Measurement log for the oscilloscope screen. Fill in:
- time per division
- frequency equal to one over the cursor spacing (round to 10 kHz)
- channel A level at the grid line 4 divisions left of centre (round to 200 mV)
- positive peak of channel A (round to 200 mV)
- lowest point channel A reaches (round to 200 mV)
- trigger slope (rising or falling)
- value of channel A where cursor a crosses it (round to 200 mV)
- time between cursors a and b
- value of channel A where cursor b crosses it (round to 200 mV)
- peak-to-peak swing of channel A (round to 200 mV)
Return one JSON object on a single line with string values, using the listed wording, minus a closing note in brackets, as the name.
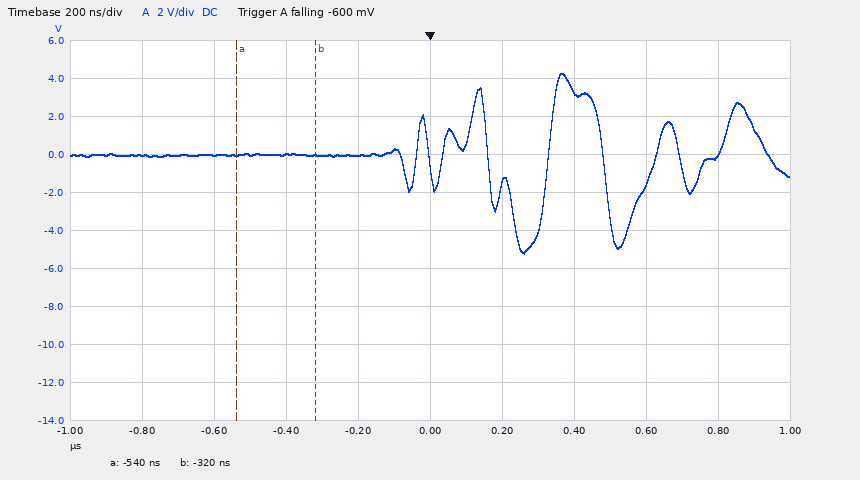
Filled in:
{"time per division": "200 ns", "frequency equal to one over the cursor spacing": "4.55 MHz", "channel A level at the grid line 4 divisions left of centre": "0.0 V", "positive peak of channel A": "4.2 V", "lowest point channel A reaches": "-5.2 V", "trigger slope": "falling", "value of channel A where cursor a crosses it": "0.0 V", "time between cursors a and b": "220 ns", "value of channel A where cursor b crosses it": "0.0 V", "peak-to-peak swing of channel A": "9.4 V"}
